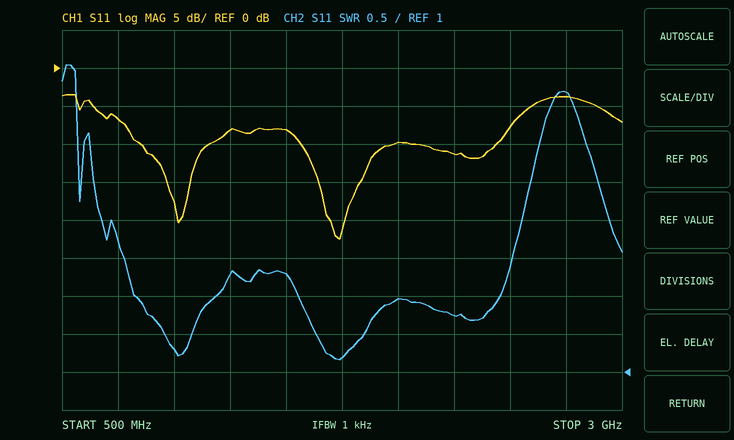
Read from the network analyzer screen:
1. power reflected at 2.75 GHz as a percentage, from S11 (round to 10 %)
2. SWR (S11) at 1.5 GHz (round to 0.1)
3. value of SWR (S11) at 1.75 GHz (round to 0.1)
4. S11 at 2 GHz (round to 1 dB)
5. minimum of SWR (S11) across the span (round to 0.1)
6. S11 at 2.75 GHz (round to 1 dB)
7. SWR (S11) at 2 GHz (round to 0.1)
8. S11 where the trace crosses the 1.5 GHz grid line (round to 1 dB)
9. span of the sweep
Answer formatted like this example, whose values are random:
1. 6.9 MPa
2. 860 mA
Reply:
1. 40 %
2. 2.3
3. 1.2
4. -10 dB
5. 1.2
6. -4 dB
7. 2.0
8. -8 dB
9. 2.5 GHz
